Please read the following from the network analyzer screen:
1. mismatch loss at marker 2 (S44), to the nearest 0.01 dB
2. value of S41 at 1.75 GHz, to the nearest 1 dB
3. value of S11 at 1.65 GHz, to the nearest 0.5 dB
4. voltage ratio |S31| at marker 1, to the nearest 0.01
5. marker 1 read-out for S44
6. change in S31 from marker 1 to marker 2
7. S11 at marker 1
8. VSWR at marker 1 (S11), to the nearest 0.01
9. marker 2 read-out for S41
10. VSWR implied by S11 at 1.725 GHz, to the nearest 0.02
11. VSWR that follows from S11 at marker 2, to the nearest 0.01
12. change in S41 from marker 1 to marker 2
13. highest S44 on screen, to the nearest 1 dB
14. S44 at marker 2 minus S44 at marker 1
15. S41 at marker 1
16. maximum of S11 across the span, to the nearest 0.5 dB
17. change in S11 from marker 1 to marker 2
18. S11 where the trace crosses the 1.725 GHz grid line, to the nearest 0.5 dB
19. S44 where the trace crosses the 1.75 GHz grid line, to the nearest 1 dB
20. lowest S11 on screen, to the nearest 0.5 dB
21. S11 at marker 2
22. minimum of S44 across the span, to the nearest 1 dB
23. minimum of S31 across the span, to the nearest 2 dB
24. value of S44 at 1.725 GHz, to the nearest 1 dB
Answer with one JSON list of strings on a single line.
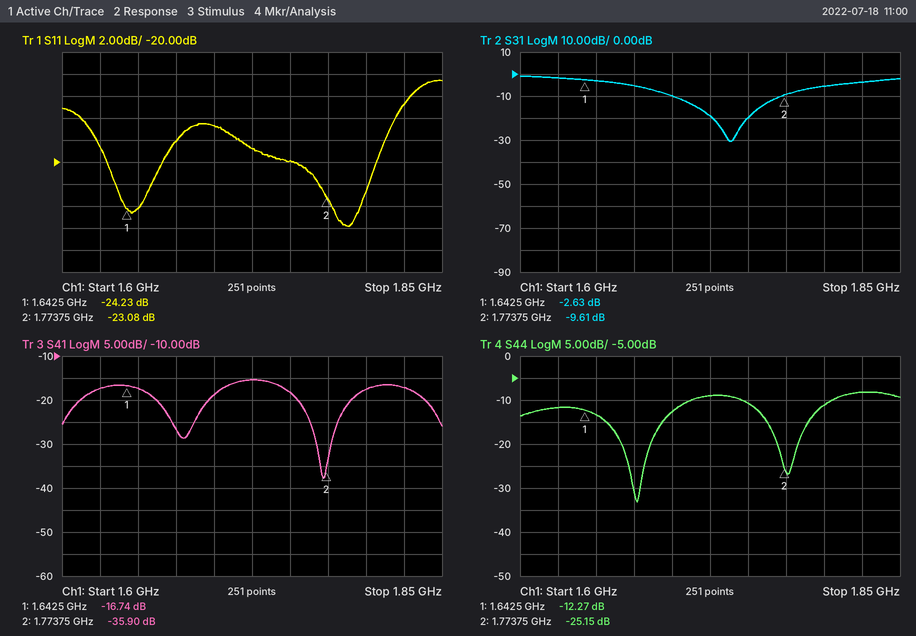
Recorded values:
["0.01 dB", "-18 dB", "-24.0 dB", "0.74", "-12.27 dB", "-6.98 dB", "-24.23 dB", "1.13", "-35.90 dB", "1.26", "1.15", "-19.16 dB", "-8 dB", "-12.88 dB", "-16.74 dB", "-12.5 dB", "1.15 dB", "-19.0 dB", "-11 dB", "-26.0 dB", "-23.08 dB", "-33 dB", "-30 dB", "-9 dB"]
